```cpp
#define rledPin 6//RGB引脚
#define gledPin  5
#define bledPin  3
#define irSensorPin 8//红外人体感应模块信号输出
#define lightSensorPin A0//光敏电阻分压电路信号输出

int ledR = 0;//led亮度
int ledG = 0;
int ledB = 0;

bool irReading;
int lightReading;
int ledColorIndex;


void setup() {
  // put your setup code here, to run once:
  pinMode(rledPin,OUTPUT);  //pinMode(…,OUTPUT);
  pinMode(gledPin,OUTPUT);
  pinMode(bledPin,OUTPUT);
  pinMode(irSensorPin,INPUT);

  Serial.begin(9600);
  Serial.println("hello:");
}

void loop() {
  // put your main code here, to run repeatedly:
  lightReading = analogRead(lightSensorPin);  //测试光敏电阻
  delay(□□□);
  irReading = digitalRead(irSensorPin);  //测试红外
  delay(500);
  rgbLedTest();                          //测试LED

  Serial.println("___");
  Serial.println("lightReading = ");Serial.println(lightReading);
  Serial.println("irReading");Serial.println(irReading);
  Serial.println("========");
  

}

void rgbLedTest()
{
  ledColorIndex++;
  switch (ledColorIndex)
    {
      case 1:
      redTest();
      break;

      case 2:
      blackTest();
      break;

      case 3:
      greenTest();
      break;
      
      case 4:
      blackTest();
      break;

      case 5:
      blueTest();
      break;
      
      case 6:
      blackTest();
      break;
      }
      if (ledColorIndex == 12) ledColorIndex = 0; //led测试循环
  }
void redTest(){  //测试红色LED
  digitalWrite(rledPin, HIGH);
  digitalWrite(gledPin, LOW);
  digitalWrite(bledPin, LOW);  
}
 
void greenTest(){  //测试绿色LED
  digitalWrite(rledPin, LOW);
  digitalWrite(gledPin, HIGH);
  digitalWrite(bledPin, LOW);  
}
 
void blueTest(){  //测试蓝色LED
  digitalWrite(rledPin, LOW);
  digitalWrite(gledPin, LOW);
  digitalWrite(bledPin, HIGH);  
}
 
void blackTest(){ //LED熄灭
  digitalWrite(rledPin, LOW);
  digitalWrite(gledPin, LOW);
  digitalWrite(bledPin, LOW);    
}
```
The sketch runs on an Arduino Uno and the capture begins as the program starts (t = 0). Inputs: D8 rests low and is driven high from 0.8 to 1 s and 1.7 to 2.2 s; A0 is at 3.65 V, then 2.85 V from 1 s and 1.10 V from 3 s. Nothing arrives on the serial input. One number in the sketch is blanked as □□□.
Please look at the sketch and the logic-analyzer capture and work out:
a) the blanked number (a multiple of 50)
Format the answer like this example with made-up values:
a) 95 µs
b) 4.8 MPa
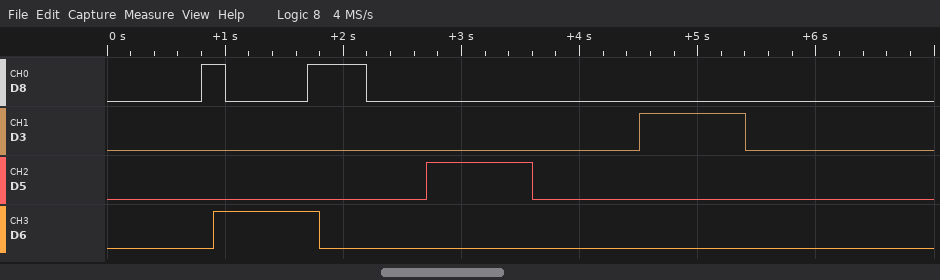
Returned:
a) 400
